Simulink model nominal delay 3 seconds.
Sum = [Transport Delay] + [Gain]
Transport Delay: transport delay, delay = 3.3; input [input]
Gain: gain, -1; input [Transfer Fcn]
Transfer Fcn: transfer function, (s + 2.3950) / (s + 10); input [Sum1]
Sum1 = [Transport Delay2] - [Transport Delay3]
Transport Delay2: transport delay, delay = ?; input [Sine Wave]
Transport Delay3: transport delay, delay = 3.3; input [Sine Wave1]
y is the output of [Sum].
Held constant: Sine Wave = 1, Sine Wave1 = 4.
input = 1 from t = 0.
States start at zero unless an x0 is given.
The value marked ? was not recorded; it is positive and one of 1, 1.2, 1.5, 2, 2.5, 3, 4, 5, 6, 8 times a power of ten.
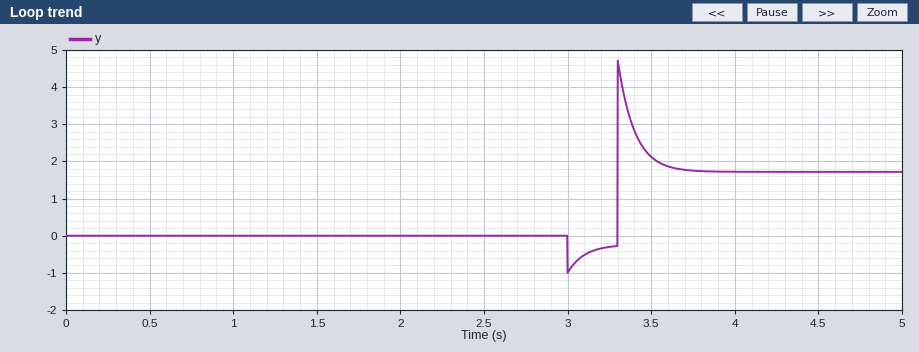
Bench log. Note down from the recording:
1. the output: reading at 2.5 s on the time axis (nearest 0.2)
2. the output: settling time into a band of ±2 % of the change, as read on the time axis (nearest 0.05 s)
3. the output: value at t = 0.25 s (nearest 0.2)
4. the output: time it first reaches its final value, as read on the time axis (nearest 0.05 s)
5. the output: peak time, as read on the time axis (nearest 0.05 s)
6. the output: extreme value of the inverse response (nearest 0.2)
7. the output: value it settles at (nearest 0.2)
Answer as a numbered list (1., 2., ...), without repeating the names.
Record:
1. 0.0
2. 3.75 s
3. 0.0
4. 3.30 s
5. 3.30 s
6. -1.0
7. 1.8
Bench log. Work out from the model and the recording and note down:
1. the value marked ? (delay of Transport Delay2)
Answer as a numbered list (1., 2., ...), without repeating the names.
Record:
1. 3
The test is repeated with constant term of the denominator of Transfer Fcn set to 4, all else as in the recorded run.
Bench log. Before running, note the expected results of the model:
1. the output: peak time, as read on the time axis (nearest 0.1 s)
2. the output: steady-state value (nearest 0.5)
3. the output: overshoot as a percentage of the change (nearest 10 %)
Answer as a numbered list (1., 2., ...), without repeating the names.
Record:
1. 3.3 s
2. 3.0
3. 50 %
